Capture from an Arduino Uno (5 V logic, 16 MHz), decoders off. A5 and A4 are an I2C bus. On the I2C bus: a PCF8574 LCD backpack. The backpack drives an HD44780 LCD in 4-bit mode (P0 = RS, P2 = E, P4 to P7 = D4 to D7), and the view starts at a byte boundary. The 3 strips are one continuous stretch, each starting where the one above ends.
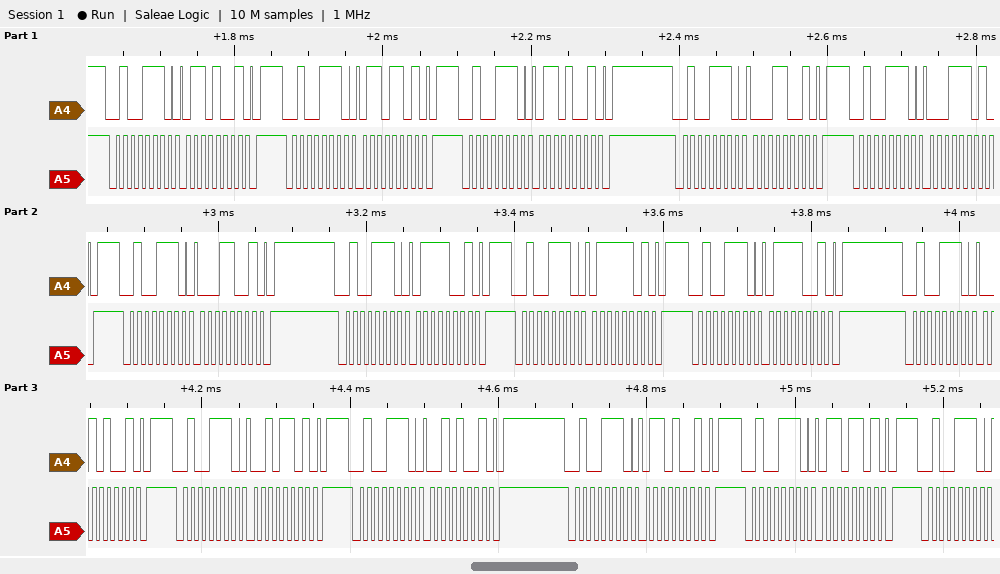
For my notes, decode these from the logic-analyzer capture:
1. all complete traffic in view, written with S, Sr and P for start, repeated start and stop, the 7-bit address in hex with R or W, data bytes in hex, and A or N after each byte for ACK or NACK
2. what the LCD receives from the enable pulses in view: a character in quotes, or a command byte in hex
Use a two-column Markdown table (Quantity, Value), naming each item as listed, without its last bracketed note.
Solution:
| Quantity | Value |
|---|---|
| all complete traffic in view, written with S, Sr and P for start, repeated start and stop, the 7-bit address in hex with R or W, data bytes in hex, and A or N after each byte for ACK or NACK | S 27W A 69 A P S 27W A 6D A P S 27W A 69 A P S 27W A 19 A P S 27W A 1D A P S 27W A 19 A P S 27W A 79 A P S 27W A 7D A P S 27W A 79 A P S 27W A 29 A P S 27W A 2D A P S 27W A 29 A P S 27W A 69 A P S 27W A 6D A P S 27W A |
| what the LCD receives from the enable pulses in view: a character in quotes, or a command byte in hex | 'a' 'r' |
